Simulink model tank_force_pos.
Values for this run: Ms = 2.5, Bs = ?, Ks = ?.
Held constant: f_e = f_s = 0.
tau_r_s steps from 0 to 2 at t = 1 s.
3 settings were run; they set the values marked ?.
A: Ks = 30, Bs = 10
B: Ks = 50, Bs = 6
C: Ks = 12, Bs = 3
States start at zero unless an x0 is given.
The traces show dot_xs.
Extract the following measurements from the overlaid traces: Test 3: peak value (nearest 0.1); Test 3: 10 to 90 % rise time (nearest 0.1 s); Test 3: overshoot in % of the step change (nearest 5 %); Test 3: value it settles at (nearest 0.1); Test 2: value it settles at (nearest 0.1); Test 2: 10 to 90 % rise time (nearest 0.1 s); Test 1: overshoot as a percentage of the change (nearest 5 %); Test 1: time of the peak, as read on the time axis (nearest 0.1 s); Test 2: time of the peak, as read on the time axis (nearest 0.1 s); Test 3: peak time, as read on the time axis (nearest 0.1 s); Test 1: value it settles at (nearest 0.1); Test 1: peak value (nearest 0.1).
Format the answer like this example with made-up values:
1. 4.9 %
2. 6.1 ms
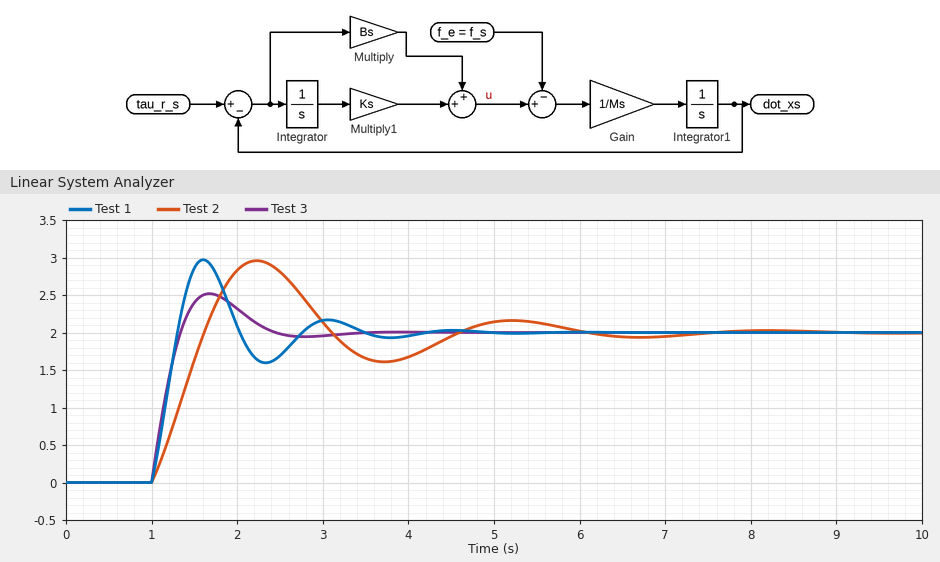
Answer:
1. 2.5
2. 0.3 s
3. 25 %
4. 2.0
5. 2.0
6. 0.5 s
7. 50 %
8. 1.6 s
9. 2.2 s
10. 1.7 s
11. 2.0
12. 3.0
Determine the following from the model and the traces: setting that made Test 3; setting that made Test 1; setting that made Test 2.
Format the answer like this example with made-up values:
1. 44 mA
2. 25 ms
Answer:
1. A
2. B
3. C
